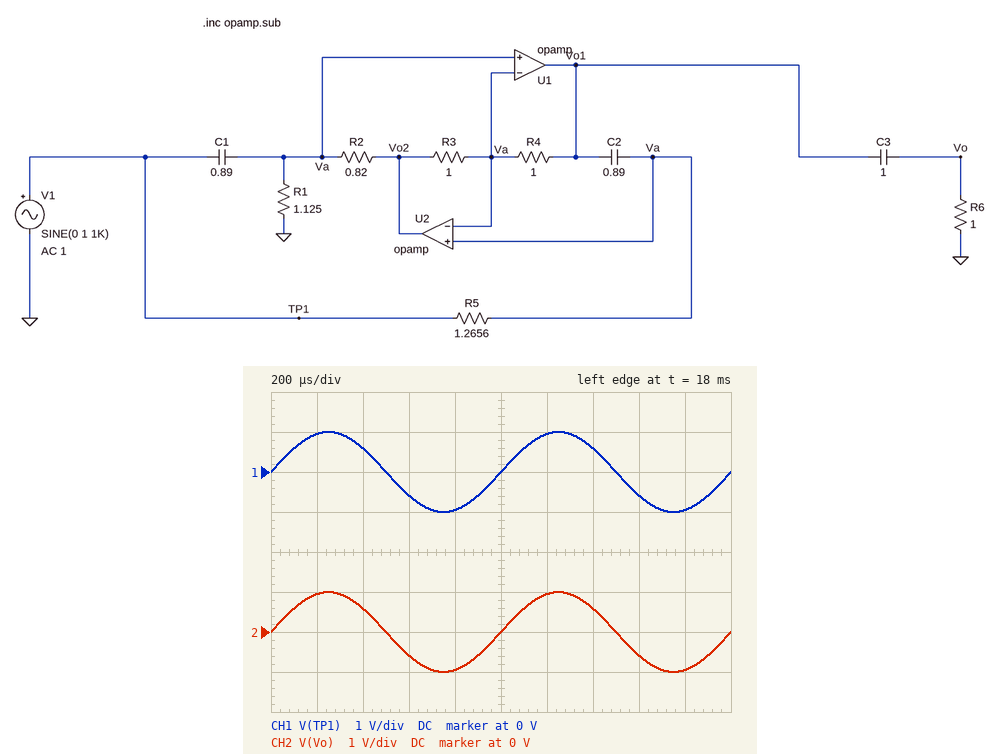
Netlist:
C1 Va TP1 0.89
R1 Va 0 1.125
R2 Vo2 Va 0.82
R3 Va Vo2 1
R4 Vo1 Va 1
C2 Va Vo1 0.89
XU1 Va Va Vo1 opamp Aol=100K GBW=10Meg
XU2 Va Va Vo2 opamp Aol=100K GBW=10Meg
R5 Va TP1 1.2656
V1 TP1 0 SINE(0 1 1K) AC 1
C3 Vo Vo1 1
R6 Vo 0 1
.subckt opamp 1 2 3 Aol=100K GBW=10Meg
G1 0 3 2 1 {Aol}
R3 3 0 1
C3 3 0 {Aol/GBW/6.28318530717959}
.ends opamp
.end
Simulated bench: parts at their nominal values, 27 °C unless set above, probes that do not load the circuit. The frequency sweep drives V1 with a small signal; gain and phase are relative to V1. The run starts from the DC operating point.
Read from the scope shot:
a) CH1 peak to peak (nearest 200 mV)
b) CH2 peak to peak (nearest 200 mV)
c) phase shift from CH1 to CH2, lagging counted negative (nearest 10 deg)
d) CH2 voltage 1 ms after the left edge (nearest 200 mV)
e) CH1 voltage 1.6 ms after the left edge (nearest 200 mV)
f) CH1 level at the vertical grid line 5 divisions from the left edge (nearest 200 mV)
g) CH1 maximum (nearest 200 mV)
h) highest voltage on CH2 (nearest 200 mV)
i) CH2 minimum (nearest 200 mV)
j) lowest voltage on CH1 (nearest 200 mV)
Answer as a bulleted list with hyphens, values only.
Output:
- 2.0 V
- 2.0 V
- 0 deg
- 0 V
- -600 mV
- 0 V
- 1.0 V
- 1.0 V
- -1.0 V
- -1.0 V
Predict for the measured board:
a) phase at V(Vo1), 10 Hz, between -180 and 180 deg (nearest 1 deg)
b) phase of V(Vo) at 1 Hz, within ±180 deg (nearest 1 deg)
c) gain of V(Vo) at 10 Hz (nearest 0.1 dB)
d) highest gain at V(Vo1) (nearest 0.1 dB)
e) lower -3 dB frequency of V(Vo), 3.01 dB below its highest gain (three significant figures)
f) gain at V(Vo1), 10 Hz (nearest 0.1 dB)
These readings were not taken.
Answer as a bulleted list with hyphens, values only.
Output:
- 6 deg
- 51 deg
- -0.1 dB
- 0 dB
- 1.13 Hz
- -0.1 dB
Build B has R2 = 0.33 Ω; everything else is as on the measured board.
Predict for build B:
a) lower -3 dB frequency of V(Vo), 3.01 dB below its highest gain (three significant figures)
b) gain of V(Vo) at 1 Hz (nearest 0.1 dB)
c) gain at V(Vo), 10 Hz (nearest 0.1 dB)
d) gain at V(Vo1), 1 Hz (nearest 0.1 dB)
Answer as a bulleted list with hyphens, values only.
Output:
- 1.14 Hz
- -3.7 dB
- -0.1 dB
- -3.6 dB
